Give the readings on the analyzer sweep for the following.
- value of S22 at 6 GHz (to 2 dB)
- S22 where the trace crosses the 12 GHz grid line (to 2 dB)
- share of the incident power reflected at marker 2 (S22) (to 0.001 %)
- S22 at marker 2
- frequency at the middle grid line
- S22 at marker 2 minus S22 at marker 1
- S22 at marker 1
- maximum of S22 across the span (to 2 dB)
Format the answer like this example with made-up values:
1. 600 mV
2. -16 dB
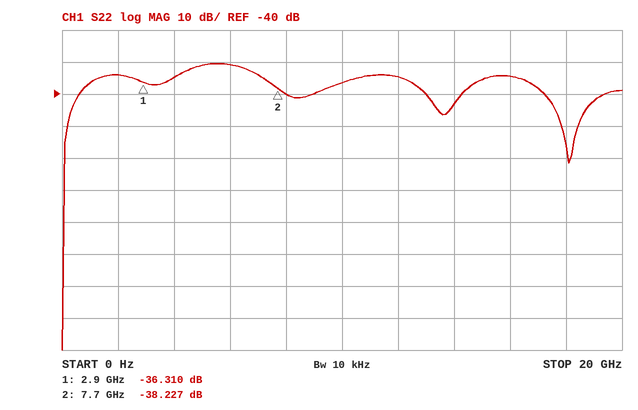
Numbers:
1. -30 dB
2. -34 dB
3. 0.015 %
4. -38.227 dB
5. 10 GHz
6. -1.917 dB
7. -36.310 dB
8. -30 dB
